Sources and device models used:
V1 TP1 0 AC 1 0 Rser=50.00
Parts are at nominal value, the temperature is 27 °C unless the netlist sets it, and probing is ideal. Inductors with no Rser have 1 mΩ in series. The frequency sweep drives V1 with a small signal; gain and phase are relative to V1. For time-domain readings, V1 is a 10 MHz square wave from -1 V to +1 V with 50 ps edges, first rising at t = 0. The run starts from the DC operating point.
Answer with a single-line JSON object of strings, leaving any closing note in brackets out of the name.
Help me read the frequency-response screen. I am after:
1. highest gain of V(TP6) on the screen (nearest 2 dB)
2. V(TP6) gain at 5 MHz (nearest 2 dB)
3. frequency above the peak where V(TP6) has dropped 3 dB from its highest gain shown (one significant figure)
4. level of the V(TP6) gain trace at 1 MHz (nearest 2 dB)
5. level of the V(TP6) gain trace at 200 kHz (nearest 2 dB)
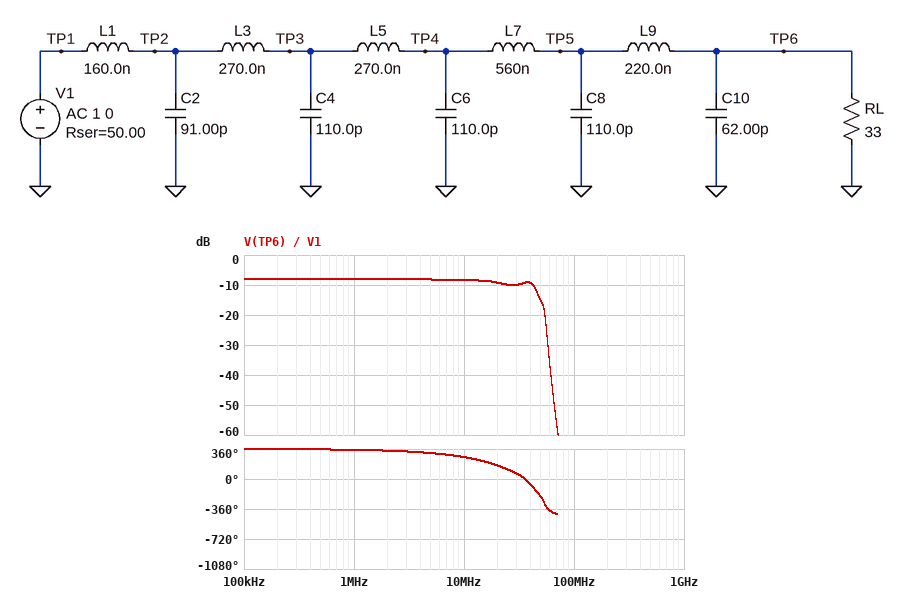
{"highest gain of V(TP6) on the screen": "-8 dB", "V(TP6) gain at 5 MHz": "-8 dB", "frequency above the peak where V(TP6) has dropped 3 dB from its highest gain shown": "40 MHz", "level of the V(TP6) gain trace at 1 MHz": "-8 dB", "level of the V(TP6) gain trace at 200 kHz": "-8 dB"}
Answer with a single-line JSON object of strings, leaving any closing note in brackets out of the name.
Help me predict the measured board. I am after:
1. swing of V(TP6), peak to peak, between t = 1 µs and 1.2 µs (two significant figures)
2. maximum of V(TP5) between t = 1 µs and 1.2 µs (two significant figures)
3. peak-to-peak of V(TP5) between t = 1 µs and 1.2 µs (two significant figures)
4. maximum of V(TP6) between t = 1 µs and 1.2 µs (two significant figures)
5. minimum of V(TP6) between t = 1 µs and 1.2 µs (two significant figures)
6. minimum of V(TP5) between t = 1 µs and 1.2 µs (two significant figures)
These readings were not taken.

{"swing of V(TP6), peak to peak, between t = 1 µs and 1.2 µs": "950 mV", "maximum of V(TP5) between t = 1 µs and 1.2 µs": "590 mV", "peak-to-peak of V(TP5) between t = 1 µs and 1.2 µs": "1.2 V", "maximum of V(TP6) between t = 1 µs and 1.2 µs": "470 mV", "minimum of V(TP6) between t = 1 µs and 1.2 µs": "-470 mV", "minimum of V(TP5) between t = 1 µs and 1.2 µs": "-590 mV"}
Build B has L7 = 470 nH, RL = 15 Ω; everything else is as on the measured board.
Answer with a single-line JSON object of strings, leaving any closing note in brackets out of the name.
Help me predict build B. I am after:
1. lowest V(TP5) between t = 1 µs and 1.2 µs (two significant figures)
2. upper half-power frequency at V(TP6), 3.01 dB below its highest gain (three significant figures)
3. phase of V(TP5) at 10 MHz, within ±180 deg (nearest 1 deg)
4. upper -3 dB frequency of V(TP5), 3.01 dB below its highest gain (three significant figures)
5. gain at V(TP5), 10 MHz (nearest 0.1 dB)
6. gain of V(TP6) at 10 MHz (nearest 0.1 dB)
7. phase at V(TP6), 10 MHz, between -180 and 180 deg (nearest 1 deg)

{"lowest V(TP5) between t = 1 µs and 1.2 µs": "-630 mV", "upper half-power frequency at V(TP6), 3.01 dB below its highest gain": "45.9 MHz", "phase of V(TP5) at 10 MHz, within ±180 deg": "-49 deg", "upper -3 dB frequency of V(TP5), 3.01 dB below its highest gain": "46.8 MHz", "gain at V(TP5), 10 MHz": "-10.8 dB", "gain of V(TP6) at 10 MHz": "-13.2 dB", "phase at V(TP6), 10 MHz, between -180 and 180 deg": "-93 deg"}
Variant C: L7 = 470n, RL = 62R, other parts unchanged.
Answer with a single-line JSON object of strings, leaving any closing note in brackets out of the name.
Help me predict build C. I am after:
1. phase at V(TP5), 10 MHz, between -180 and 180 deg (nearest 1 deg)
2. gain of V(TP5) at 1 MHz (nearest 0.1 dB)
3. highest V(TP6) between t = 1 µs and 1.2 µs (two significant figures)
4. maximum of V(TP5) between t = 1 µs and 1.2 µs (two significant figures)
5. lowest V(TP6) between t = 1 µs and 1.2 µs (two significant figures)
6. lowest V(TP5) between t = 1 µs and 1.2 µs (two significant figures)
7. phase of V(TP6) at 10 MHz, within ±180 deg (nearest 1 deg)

{"phase at V(TP5), 10 MHz, between -180 and 180 deg": "-81 deg", "gain of V(TP5) at 1 MHz": "-5.1 dB", "highest V(TP6) between t = 1 µs and 1.2 µs": "720 mV", "maximum of V(TP5) between t = 1 µs and 1.2 µs": "640 mV", "lowest V(TP6) between t = 1 µs and 1.2 µs": "-720 mV", "lowest V(TP5) between t = 1 µs and 1.2 µs": "-640 mV", "phase of V(TP6) at 10 MHz, within ±180 deg": "-94 deg"}
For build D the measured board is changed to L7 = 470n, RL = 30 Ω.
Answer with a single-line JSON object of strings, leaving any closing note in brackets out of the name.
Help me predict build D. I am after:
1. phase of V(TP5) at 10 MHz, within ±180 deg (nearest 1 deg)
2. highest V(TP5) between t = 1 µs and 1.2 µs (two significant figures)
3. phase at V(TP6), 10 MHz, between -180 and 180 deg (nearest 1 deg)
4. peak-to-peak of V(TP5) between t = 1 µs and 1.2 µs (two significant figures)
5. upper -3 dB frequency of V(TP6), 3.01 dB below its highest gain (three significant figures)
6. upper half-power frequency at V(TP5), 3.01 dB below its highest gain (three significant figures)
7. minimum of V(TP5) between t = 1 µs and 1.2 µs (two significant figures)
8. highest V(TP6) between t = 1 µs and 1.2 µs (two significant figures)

{"phase of V(TP5) at 10 MHz, within ±180 deg": "-68 deg", "highest V(TP5) between t = 1 µs and 1.2 µs": "640 mV", "phase at V(TP6), 10 MHz, between -180 and 180 deg": "-94 deg", "peak-to-peak of V(TP5) between t = 1 µs and 1.2 µs": "1.3 V", "upper -3 dB frequency of V(TP6), 3.01 dB below its highest gain": "47.2 MHz", "upper half-power frequency at V(TP5), 3.01 dB below its highest gain": "50.0 MHz", "minimum of V(TP5) between t = 1 µs and 1.2 µs": "-640 mV", "highest V(TP6) between t = 1 µs and 1.2 µs": "480 mV"}
